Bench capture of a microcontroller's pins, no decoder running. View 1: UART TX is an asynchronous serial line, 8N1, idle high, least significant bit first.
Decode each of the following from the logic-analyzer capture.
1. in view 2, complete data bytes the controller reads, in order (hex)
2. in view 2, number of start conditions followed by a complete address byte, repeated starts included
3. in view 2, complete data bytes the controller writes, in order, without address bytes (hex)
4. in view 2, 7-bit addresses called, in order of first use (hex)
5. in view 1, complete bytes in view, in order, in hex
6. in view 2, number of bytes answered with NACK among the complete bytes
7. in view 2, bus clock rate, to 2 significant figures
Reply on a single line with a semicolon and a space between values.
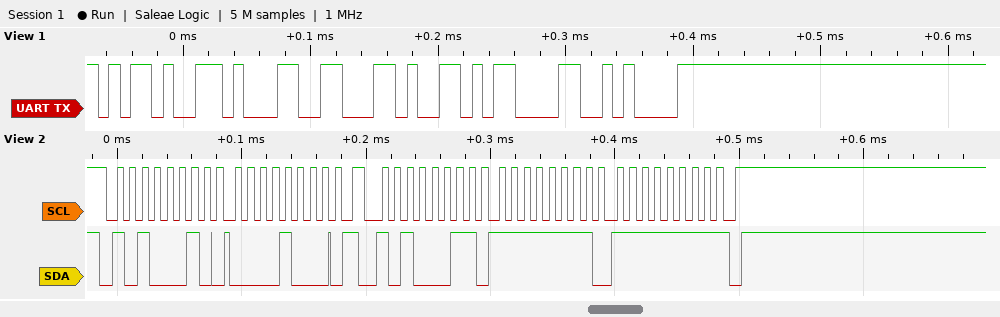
FF FF; 2; 08; 0x51; 0x2D 0x31 0x2C 0x0D 0x0A; 1; 100 kHz
